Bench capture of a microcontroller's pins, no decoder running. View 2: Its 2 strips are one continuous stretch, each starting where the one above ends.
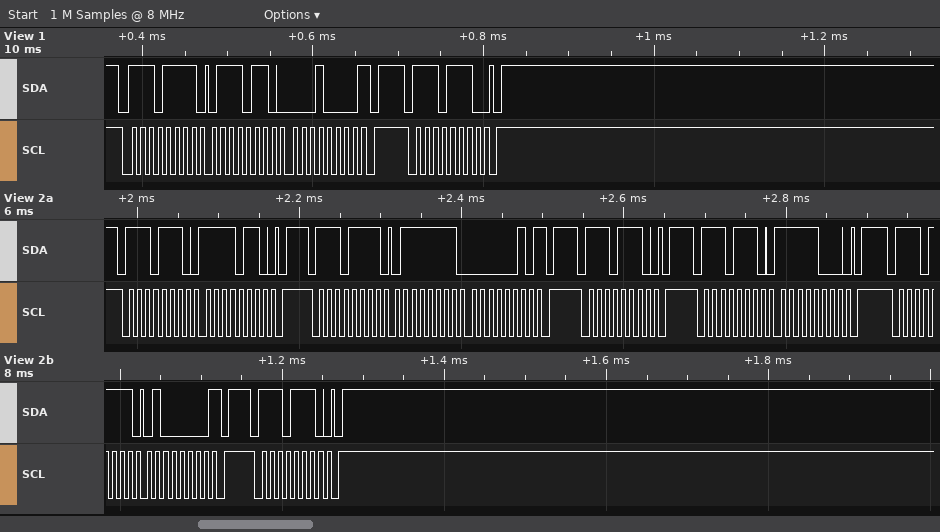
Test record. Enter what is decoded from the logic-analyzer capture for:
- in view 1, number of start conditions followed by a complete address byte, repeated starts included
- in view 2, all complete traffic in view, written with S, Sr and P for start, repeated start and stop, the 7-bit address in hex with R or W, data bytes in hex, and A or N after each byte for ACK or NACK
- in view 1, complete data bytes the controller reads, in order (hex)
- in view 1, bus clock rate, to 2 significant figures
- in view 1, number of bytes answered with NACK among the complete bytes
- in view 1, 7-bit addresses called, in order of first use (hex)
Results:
2
S 77W A F6 A P S 77R A 7F A 02 N P S 77W A P S 77W A F8 A P S 77R A 40 N P S 77W A P
76 10
100 kHz
1
0x77
